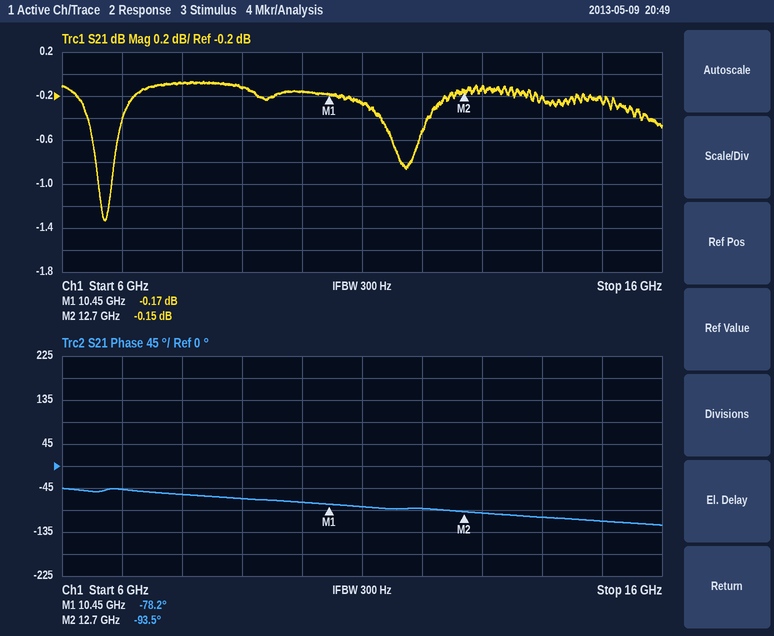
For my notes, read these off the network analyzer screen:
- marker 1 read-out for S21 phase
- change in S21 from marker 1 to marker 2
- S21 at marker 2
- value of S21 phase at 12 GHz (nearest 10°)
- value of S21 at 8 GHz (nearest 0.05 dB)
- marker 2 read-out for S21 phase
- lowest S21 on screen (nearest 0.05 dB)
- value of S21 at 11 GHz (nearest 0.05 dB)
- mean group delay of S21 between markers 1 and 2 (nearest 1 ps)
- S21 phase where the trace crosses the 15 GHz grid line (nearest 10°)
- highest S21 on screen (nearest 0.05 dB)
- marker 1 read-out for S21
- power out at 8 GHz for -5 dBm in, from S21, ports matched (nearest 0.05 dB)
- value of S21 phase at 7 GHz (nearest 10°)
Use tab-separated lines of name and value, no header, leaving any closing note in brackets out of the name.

marker 1 read-out for S21 phase	-78.2°
change in S21 from marker 1 to marker 2	0.02 dB
S21 at marker 2	-0.15 dB
value of S21 phase at 12 GHz	-90°
value of S21 at 8 GHz	-0.10 dB
marker 2 read-out for S21 phase	-93.5°
lowest S21 on screen	-1.35 dB
value of S21 at 11 GHz	-0.25 dB
mean group delay of S21 between markers 1 and 2	19 ps
S21 phase where the trace crosses the 15 GHz grid line	-110°
highest S21 on screen	-0.05 dB
marker 1 read-out for S21	-0.17 dB
power out at 8 GHz for -5 dBm in, from S21, ports matched	-5.10 dBm
value of S21 phase at 7 GHz	-50°
